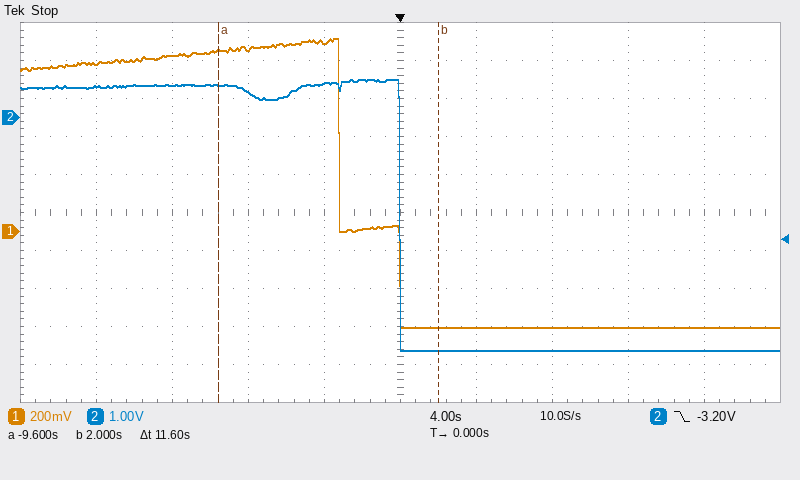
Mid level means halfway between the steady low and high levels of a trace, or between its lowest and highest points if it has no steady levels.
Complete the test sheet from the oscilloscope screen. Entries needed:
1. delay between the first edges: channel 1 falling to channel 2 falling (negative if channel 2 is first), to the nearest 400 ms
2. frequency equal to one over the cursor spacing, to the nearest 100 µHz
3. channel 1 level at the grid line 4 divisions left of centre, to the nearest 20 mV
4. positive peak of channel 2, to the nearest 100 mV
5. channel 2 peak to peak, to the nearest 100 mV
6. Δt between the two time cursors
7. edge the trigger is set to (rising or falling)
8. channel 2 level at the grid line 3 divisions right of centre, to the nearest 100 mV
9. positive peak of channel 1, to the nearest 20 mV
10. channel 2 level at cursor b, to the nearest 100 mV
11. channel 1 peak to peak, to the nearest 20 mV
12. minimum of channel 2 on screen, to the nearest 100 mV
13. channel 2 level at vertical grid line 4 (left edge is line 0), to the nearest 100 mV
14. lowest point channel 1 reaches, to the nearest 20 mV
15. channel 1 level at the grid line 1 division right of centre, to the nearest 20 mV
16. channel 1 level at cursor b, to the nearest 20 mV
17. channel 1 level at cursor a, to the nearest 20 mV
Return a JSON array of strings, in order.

["+3.2 s", "86.2 mHz", "880 mV", "1.0 V", "7.1 V", "11.6 s", "falling", "-6.1 V", "1.02 V", "-6.1 V", "1.52 V", "-6.1 V", "900 mV", "-500 mV", "-500 mV", "-500 mV", "960 mV"]
